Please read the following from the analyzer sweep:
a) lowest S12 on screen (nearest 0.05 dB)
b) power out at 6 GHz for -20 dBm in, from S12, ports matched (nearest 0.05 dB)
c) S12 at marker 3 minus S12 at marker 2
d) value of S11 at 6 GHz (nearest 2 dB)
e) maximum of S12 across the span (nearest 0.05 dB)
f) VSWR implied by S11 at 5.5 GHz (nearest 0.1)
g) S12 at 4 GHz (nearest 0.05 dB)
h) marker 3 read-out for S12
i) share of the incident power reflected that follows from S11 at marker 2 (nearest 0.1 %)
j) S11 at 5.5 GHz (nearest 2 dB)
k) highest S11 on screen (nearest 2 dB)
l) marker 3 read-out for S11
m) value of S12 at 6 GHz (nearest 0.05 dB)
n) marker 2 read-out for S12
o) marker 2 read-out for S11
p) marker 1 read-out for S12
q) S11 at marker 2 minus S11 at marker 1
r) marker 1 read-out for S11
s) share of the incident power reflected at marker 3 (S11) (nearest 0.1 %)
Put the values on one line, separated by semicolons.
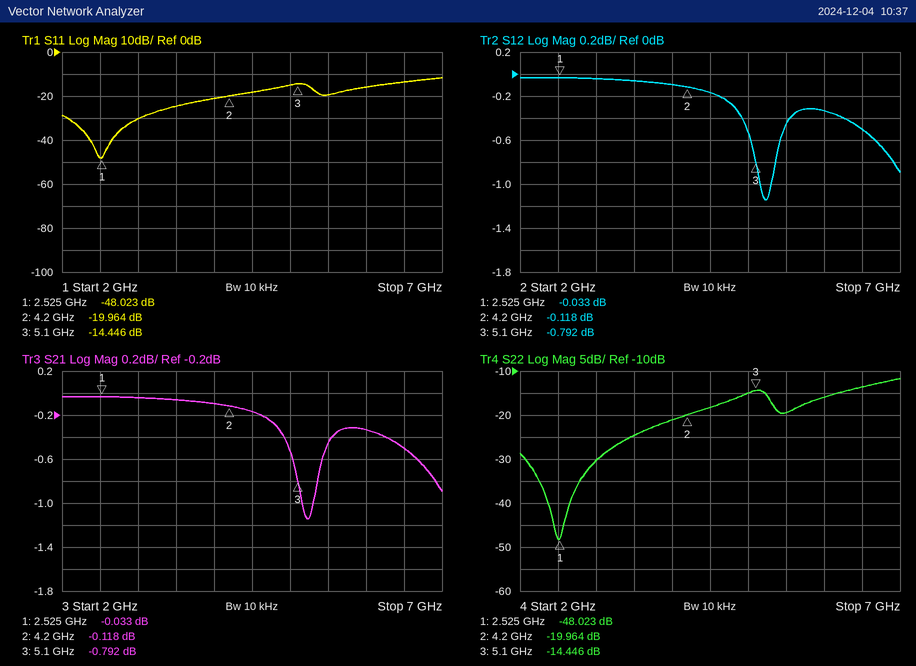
-1.15 dB; -20.35 dBm; -0.674 dB; -16 dB; -0.05 dB; 1.2; -0.10 dB; -0.792 dB; 1.0 %; -20 dB; -12 dB; -14.446 dB; -0.35 dB; -0.118 dB; -19.964 dB; -0.033 dB; 28.059 dB; -48.023 dB; 3.6 %
